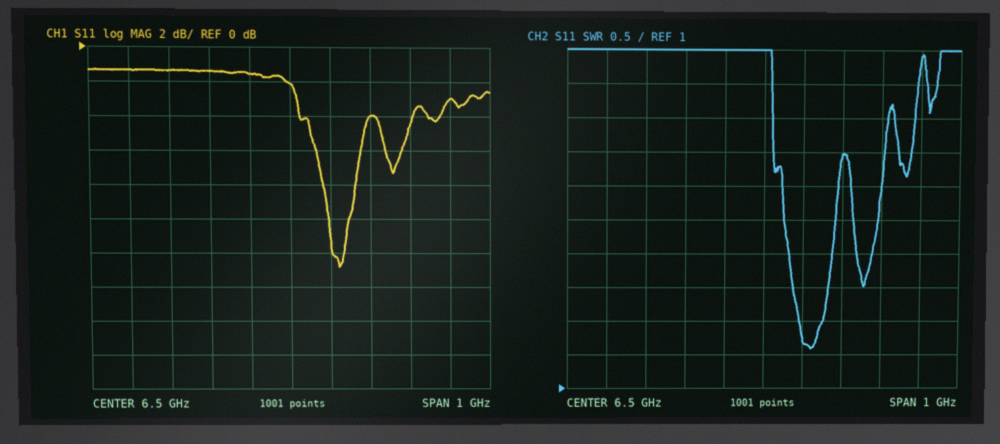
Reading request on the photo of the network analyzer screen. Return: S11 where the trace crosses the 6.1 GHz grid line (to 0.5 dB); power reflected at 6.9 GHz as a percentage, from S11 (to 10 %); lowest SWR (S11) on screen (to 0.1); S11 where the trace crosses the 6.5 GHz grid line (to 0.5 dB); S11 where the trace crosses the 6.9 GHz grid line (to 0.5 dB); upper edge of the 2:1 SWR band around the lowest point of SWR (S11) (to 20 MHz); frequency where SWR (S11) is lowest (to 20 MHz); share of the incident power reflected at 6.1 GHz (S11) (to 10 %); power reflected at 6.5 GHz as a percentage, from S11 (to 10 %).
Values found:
-1.5 dB
50 %
1.6
-2.0 dB
-3.0 dB
6.66 GHz
6.62 GHz
70 %
60 %
